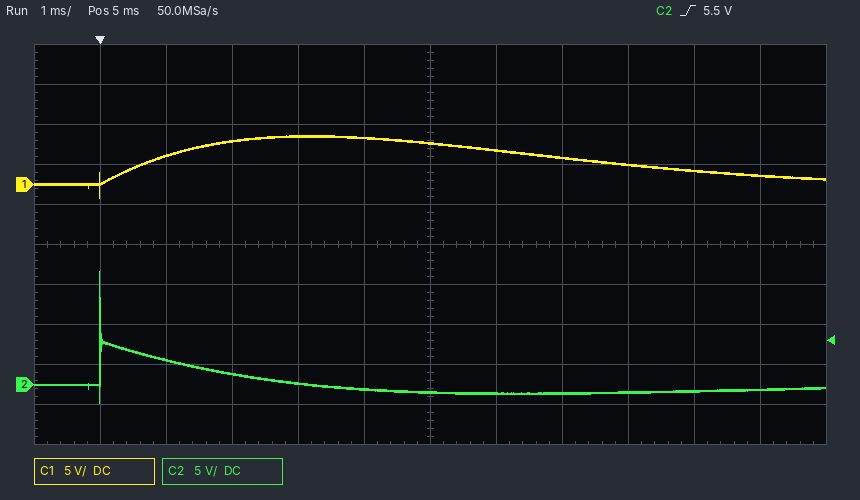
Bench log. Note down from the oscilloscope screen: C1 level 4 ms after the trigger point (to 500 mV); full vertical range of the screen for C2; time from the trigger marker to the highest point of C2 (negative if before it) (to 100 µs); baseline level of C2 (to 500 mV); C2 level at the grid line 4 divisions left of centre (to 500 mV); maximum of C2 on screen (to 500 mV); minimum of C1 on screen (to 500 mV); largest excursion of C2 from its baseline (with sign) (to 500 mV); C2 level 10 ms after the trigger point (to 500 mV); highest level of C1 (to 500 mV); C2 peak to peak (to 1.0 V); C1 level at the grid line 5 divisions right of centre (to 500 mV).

6.0 V
50 V
0.0 ms
-1.0 V
3.0 V
14.0 V
-1.5 V
+15.0 V
-500 mV
6.0 V
16.0 V
1.0 V
